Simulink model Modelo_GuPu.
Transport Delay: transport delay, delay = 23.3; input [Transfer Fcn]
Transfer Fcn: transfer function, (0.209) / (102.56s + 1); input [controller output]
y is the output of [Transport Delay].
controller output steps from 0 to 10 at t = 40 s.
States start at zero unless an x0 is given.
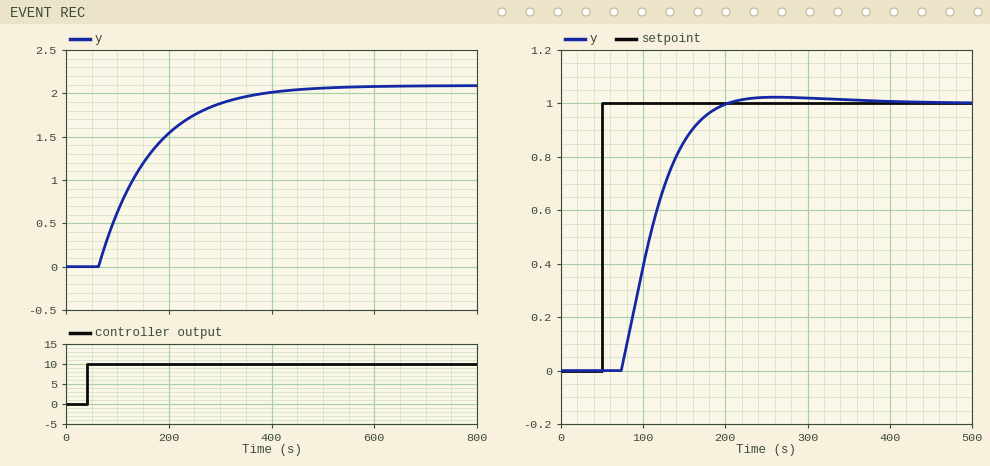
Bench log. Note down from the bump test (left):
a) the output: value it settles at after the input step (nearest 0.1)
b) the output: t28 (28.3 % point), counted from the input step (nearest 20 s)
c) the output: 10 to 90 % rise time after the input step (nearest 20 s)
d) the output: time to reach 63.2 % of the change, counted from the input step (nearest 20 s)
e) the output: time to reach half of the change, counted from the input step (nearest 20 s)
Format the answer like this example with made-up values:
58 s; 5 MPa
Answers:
2.1; 60 s; 220 s; 120 s; 100 s
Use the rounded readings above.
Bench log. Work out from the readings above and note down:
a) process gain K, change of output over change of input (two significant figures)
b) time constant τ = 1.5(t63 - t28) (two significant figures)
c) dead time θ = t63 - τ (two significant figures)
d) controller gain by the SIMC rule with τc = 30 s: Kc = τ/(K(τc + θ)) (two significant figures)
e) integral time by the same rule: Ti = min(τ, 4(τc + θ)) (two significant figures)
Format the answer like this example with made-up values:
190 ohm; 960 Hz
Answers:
0.21; 90 s; 30 s; 7.1; 90 s
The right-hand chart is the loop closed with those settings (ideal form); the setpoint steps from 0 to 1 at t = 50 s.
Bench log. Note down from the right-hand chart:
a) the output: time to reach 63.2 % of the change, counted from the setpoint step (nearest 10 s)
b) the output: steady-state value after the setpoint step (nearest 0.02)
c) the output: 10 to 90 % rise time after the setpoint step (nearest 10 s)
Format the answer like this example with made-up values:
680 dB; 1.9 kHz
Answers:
70 s; 1.00; 80 s
